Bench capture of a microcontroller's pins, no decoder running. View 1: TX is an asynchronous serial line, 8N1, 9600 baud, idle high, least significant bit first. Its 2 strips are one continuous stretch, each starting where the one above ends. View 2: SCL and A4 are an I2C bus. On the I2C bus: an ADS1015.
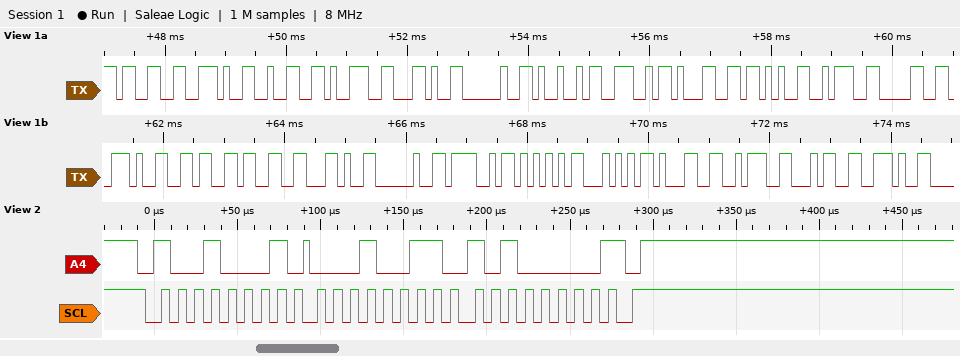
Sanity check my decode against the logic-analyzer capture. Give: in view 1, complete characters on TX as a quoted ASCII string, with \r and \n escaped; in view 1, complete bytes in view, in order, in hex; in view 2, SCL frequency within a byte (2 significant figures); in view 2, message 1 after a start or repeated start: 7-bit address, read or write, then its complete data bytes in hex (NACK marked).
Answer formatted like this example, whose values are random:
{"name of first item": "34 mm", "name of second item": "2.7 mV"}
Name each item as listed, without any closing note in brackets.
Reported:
{"in view 1, complete characters on TX as a quoted ASCII string, with \\r and \\n escaped": "\"3.29, IN1+:0.63, OUT1:4.\"", "in view 1, complete bytes in view, in order, in hex": "33 2E 32 39 2C 20 49 4E 31 2B 3A 30 2E 36 33 2C 20 4F 55 54 31 3A 34 2E", "in view 2, SCL frequency within a byte": "100 kHz", "in view 2, message 1 after a start or repeated start: 7-bit address, read or write, then its complete data bytes in hex": "0x48 read: 13 A0 NACK"}
